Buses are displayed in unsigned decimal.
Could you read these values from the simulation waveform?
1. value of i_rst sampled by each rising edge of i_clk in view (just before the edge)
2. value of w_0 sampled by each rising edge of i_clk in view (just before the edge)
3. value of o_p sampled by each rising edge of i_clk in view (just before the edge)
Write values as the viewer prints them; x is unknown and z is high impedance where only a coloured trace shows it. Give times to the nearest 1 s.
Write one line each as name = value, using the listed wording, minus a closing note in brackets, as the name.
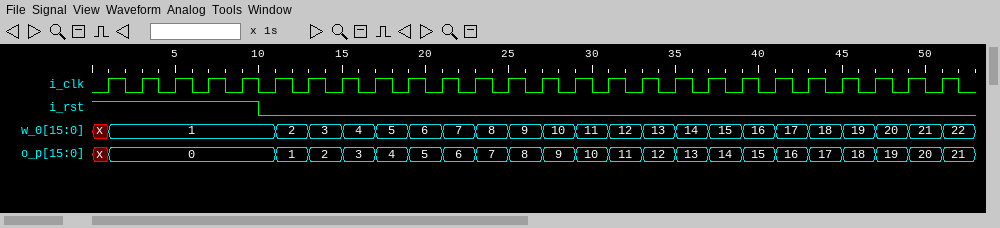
value of i_rst sampled by each rising edge of i_clk in view = 1 1 1 1 1 0 0 0 0 0 0 0 0 0 0 0 0 0 0 0 0 0 0 0 0 0
value of w_0 sampled by each rising edge of i_clk in view = x, 1, 1, 1, 1, 1, 2, 3, 4, 5, 6, 7, 8, 9, 10, 11, 12, 13, 14, 15, 16, 17, 18, 19, 20, 21
value of o_p sampled by each rising edge of i_clk in view = x, 0, 0, 0, 0, 0, 1, 2, 3, 4, 5, 6, 7, 8, 9, 10, 11, 12, 13, 14, 15, 16, 17, 18, 19, 20
